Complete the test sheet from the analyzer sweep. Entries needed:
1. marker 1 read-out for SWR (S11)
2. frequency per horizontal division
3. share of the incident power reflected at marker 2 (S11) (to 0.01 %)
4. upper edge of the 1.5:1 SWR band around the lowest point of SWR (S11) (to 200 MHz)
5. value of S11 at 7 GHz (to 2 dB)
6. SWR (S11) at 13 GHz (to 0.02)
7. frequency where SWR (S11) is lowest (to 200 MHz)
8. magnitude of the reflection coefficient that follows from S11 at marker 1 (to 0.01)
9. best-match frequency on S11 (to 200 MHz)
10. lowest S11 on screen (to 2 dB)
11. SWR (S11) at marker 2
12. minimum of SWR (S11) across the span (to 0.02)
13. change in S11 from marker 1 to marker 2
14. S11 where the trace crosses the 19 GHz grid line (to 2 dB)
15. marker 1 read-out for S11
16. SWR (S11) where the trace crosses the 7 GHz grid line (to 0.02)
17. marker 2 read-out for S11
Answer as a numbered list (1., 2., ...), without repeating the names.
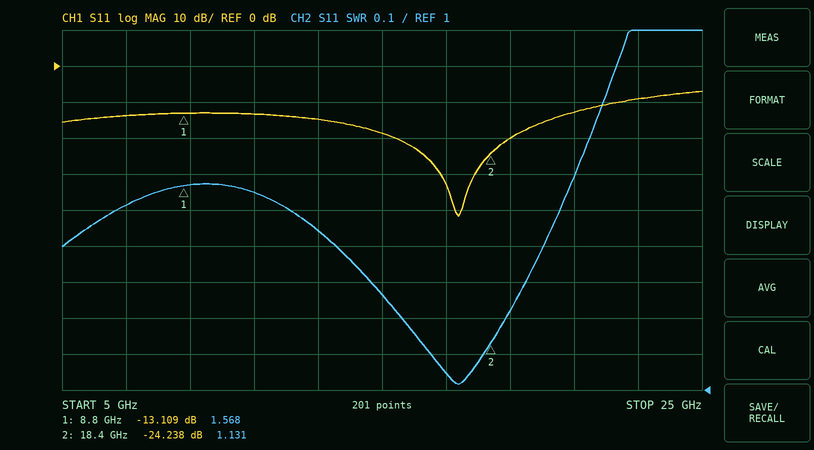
1. 1.568
2. 2 GHz
3. 0.38 %
4. 20.6 GHz
5. -14 dB
6. 1.44
7. 17.4 GHz
8. 0.22
9. 17.4 GHz
10. -42 dB
11. 1.131
12. 1.02
13. -11.129 dB
14. -20 dB
15. -13.109 dB
16. 1.52
17. -24.238 dB
